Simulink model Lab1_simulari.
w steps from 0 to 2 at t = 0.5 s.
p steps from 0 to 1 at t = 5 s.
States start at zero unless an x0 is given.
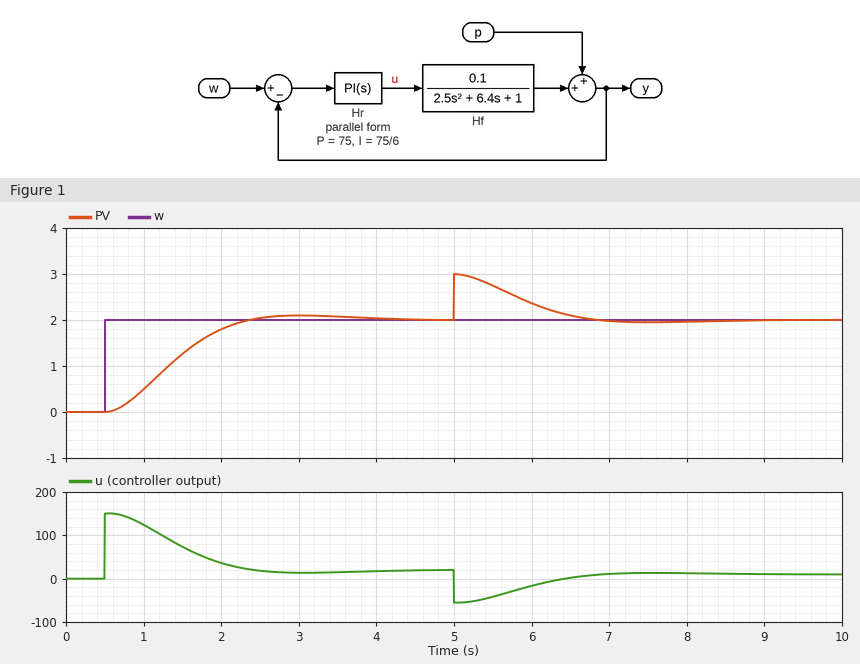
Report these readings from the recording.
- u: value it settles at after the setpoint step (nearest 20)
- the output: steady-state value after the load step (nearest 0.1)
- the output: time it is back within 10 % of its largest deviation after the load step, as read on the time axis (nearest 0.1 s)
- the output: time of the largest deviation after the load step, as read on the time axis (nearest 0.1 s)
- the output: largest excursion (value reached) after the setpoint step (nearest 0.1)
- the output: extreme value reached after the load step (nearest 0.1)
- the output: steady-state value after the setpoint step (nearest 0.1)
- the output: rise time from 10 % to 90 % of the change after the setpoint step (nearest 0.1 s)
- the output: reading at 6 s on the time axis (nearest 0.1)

20
2.0
6.5 s
5.0 s
2.1
3.0
2.0
1.2 s
2.4
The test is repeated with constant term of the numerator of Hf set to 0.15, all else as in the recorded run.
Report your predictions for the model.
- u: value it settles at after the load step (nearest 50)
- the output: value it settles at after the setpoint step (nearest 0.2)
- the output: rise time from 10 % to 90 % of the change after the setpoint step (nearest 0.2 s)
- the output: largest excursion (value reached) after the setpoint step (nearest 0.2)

0
2.0
0.8 s
2.2
